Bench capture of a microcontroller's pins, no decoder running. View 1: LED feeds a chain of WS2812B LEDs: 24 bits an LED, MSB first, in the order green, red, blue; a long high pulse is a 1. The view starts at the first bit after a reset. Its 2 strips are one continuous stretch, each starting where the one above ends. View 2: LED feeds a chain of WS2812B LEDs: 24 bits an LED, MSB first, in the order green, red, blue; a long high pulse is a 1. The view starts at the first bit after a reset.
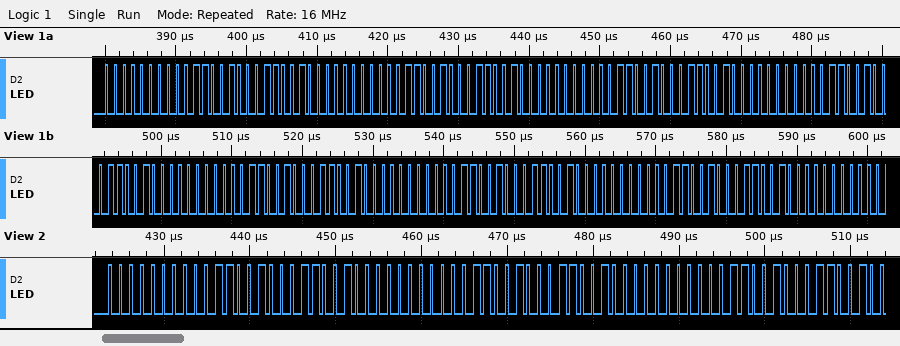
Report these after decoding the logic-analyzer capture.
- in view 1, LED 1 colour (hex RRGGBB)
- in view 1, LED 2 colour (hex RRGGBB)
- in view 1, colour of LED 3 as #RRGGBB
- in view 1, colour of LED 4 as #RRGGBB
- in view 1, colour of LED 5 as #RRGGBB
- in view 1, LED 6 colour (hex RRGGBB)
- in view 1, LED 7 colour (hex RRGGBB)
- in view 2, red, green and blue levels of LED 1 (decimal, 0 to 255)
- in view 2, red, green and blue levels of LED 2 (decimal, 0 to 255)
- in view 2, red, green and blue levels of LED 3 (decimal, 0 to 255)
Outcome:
#320032
#320032
#320032
#320032
#320032
#320032
#320032
50, 0, 50
50, 0, 50
50, 0, 50
